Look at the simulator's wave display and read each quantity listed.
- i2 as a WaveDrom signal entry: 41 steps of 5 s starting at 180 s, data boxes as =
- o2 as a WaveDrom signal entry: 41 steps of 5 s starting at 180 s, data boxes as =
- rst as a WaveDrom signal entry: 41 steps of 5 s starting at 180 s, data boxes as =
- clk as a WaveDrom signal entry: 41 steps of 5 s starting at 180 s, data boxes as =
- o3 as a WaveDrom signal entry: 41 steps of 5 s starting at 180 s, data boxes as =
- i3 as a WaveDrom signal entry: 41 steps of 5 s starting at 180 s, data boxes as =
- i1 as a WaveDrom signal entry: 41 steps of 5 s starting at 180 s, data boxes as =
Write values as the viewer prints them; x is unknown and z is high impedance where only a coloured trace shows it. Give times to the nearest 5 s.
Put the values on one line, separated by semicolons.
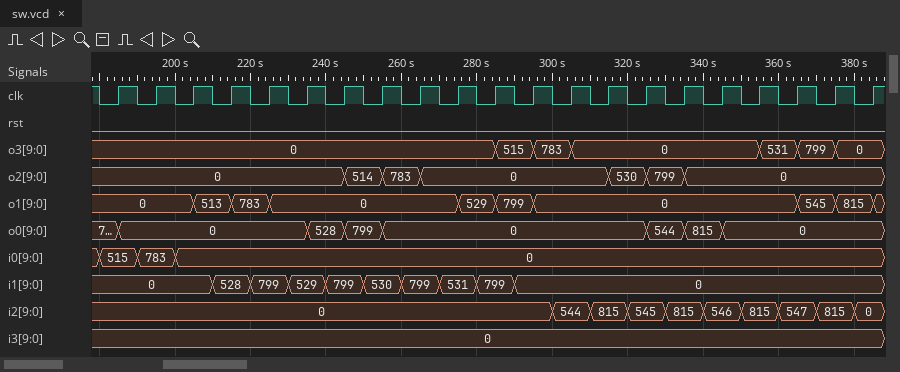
{name: 'i2', wave: '=.......................=.=.=.=.=.=.=.=.=', data: '0 544 815 545 815 546 815 547 815 0'}; {name: 'o2', wave: '=............=.=.=.........=.=.=.........', data: '0 514 783 0 530 799 0'}; {name: 'rst', wave: '0........................................'}; {name: 'clk', wave: '01010101010101010101010101010101010101010'}; {name: 'o3', wave: '=....................=.=.=.........=.=.=.', data: '0 515 783 0 531 799 0'}; {name: 'i3', wave: '=........................................', data: '0'}; {name: 'i1', wave: '=.....=.=.=.=.=.=.=.=.=..................', data: '0 528 799 529 799 530 799 531 799 0'}
